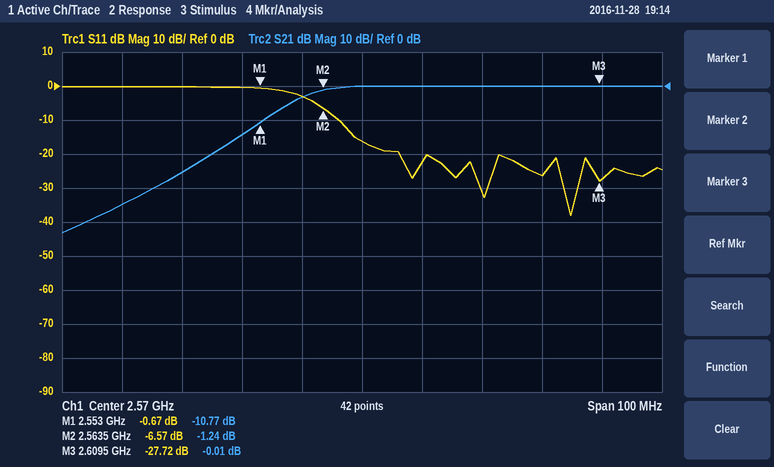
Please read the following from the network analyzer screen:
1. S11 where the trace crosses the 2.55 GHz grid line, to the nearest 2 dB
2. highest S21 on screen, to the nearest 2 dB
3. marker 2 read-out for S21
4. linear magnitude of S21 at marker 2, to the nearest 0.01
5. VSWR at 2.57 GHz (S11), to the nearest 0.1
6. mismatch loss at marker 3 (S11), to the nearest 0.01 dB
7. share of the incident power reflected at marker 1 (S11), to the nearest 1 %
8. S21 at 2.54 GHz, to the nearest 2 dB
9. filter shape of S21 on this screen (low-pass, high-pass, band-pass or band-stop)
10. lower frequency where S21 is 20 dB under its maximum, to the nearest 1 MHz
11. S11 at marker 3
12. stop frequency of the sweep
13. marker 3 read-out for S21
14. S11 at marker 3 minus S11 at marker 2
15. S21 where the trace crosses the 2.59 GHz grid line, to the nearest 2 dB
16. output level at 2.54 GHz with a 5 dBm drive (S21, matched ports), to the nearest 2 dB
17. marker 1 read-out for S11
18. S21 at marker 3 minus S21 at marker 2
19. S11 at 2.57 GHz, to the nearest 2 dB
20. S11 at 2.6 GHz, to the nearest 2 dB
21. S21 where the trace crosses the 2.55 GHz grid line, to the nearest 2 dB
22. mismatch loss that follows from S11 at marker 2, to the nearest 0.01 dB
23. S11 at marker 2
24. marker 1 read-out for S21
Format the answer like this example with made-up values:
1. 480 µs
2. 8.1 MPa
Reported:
1. 0 dB
2. 0 dB
3. -1.24 dB
4. 0.87
5. 1.4
6. 0.01 dB
7. 86 %
8. -26 dB
9. high-pass
10. 2.545 GHz
11. -27.72 dB
12. 2.62 GHz
13. -0.01 dB
14. -21.15 dB
15. 0 dB
16. -20 dBm
17. -0.67 dB
18. 1.23 dB
19. -16 dB
20. -26 dB
21. -14 dB
22. 1.08 dB
23. -6.57 dB
24. -10.77 dB
